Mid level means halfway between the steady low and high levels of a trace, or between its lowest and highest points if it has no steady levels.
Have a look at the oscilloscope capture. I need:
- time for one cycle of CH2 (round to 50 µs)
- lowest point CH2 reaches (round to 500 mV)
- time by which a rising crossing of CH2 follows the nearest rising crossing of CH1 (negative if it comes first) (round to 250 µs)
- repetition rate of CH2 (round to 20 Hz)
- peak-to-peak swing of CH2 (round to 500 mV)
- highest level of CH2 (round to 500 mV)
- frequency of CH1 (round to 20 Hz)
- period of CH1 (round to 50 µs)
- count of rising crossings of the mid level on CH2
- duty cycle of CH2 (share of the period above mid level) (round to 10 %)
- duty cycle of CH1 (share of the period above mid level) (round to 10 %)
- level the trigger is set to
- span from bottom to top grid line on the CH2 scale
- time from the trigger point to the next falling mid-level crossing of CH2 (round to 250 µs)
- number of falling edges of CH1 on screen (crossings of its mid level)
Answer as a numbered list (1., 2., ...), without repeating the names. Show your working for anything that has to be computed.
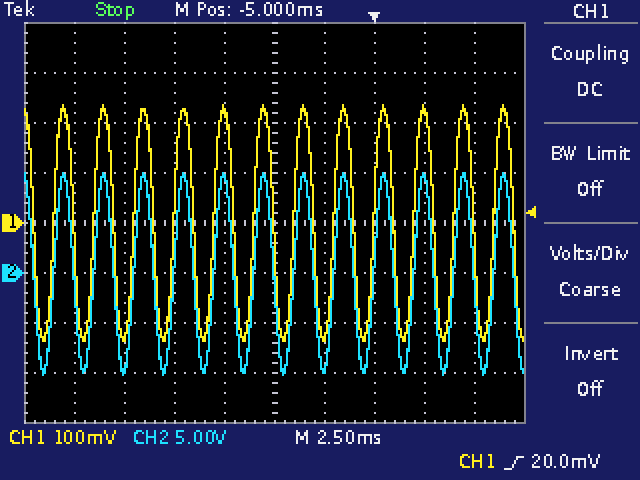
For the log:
1. 2.00 ms
2. -10.0 V
3. 0.00 ms
4. 1 / 2.00 ms ≈ 500 Hz
5. 10.0 V − (-10.0 V) = 20.0 V
6. 10.0 V
7. 1 / 2.00 ms ≈ 500 Hz
8. 2.00 ms
9. 12
10. 50 %
11. 50 %
12. 20.0 mV
13. 40 V
14. 1.00 ms
15. 13
